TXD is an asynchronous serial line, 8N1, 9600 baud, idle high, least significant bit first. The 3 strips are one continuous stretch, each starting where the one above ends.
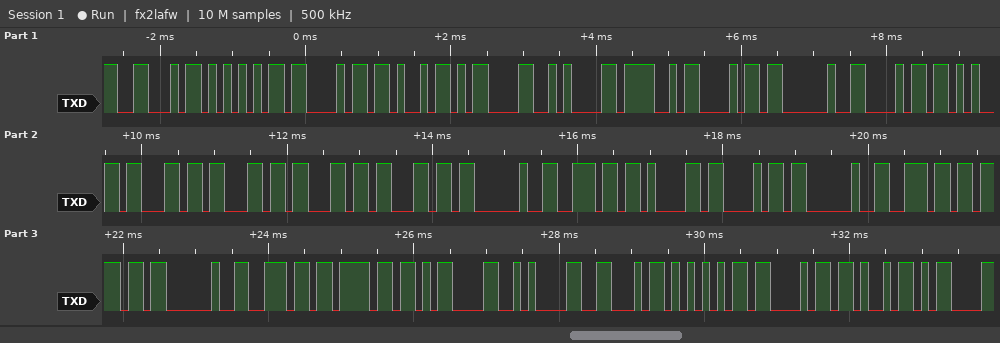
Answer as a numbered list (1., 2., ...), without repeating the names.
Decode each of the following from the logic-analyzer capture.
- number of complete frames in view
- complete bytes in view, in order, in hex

1. 32
2. 0x46 0x55 0x43 0x4B 0x0D 0x0A 0x4F 0x68 0x20 0x68 0x65 0x6C 0x6C 0x6C 0x6C 0x20 0x6E 0x61 0x68 0x20 0x6E 0x6F 0x20 0x6E 0x6F 0x0D 0x0A 0x46 0x55 0x43 0x4B 0x0D
